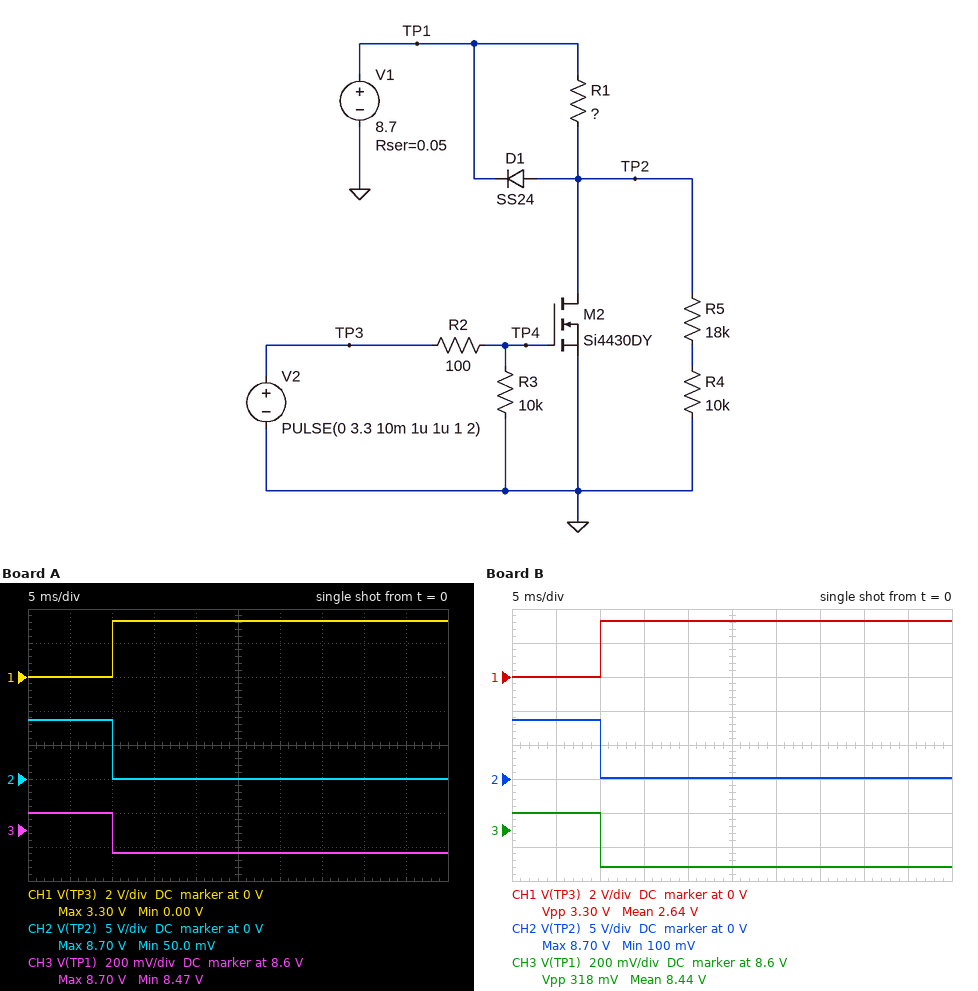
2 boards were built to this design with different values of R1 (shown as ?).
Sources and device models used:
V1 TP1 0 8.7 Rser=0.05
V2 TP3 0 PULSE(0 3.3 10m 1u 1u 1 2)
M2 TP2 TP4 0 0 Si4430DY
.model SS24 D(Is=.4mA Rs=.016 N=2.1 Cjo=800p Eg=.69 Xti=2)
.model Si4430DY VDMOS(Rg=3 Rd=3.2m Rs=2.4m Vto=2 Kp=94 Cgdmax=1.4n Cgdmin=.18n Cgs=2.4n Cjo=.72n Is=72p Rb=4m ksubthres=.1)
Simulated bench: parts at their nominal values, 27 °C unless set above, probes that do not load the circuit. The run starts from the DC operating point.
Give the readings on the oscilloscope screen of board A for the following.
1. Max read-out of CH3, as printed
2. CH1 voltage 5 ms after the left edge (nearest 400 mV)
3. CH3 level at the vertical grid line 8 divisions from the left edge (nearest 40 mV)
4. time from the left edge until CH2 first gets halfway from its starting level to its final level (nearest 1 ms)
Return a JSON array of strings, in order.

["8.70 V", "0 V", "8.48 V", "10 ms"]
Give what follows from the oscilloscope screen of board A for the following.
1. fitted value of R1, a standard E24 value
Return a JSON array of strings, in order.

["1.8 Ω"]
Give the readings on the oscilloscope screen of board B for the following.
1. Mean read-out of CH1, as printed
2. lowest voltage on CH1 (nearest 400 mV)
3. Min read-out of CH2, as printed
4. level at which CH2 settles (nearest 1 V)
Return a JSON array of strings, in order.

["2.64 V", "0 V", "100 mV", "0 V"]
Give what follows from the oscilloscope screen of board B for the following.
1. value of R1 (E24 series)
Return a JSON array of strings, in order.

["1.3 Ω"]
